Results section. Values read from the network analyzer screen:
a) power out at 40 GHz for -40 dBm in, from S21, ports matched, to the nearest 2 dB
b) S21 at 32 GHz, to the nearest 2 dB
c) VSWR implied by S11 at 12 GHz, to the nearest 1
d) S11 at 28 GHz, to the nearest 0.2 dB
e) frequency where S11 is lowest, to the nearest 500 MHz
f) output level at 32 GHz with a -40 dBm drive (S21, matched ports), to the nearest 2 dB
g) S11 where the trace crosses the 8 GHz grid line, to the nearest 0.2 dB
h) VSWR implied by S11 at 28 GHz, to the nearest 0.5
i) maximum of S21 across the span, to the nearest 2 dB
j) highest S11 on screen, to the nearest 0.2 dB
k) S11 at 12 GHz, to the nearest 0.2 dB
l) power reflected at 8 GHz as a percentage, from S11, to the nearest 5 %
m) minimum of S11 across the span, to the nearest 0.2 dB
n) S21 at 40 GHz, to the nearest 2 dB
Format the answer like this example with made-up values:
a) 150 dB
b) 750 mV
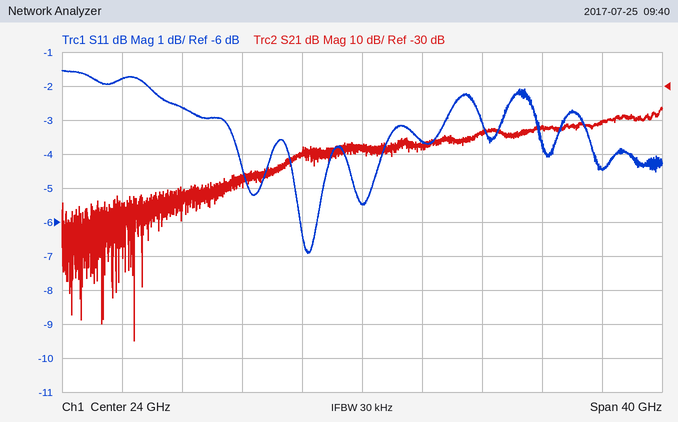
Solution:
a) -80 dBm
b) -44 dB
c) 7
d) -3.6 dB
e) 20.5 GHz
f) -84 dBm
g) -1.8 dB
h) 5.0
i) -36 dB
j) -1.6 dB
k) -2.6 dB
l) 65 %
m) -7.0 dB
n) -40 dB
